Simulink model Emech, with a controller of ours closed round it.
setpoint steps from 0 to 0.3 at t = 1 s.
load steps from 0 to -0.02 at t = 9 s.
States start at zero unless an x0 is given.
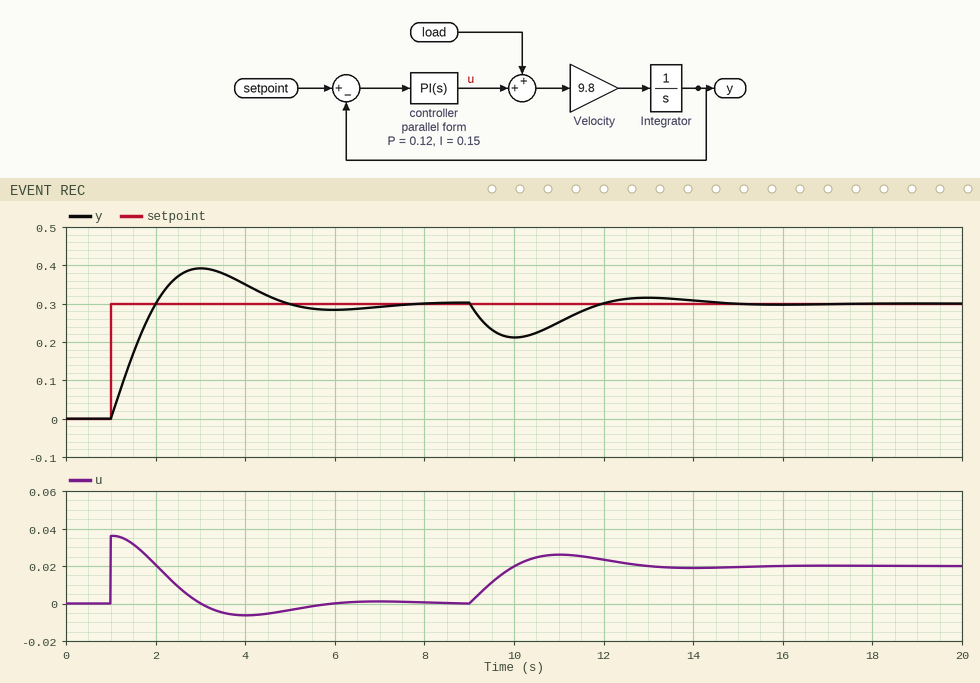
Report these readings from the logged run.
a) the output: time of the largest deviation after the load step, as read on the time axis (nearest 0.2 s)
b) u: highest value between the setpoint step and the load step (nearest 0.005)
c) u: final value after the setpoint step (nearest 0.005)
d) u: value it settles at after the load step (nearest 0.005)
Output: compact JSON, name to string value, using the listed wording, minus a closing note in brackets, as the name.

{"the output: time of the largest deviation after the load step, as read on the time axis": "10.0 s", "u: highest value between the setpoint step and the load step": "0.035", "u: final value after the setpoint step": "0.000", "u: value it settles at after the load step": "0.020"}
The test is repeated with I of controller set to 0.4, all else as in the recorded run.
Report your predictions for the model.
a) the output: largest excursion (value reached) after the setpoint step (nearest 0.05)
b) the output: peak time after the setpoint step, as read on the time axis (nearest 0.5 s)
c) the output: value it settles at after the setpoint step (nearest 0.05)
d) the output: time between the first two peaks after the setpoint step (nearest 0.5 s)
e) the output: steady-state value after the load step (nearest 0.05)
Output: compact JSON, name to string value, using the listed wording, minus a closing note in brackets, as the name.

{"the output: largest excursion (value reached) after the setpoint step": "0.45", "the output: peak time after the setpoint step, as read on the time axis": "2.5 s", "the output: value it settles at after the setpoint step": "0.30", "the output: time between the first two peaks after the setpoint step": "3.5 s", "the output: steady-state value after the load step": "0.30"}
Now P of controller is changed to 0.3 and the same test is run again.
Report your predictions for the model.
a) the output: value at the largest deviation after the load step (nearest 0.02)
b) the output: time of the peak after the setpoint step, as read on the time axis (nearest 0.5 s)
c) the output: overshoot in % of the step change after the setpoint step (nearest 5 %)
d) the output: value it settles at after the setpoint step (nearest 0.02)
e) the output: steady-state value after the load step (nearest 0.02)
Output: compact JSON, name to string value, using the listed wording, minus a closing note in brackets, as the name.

{"the output: value at the largest deviation after the load step": "0.24", "the output: time of the peak after the setpoint step, as read on the time axis": "2.5 s", "the output: overshoot in % of the step change after the setpoint step": "10 %", "the output: value it settles at after the setpoint step": "0.30", "the output: steady-state value after the load step": "0.30"}
